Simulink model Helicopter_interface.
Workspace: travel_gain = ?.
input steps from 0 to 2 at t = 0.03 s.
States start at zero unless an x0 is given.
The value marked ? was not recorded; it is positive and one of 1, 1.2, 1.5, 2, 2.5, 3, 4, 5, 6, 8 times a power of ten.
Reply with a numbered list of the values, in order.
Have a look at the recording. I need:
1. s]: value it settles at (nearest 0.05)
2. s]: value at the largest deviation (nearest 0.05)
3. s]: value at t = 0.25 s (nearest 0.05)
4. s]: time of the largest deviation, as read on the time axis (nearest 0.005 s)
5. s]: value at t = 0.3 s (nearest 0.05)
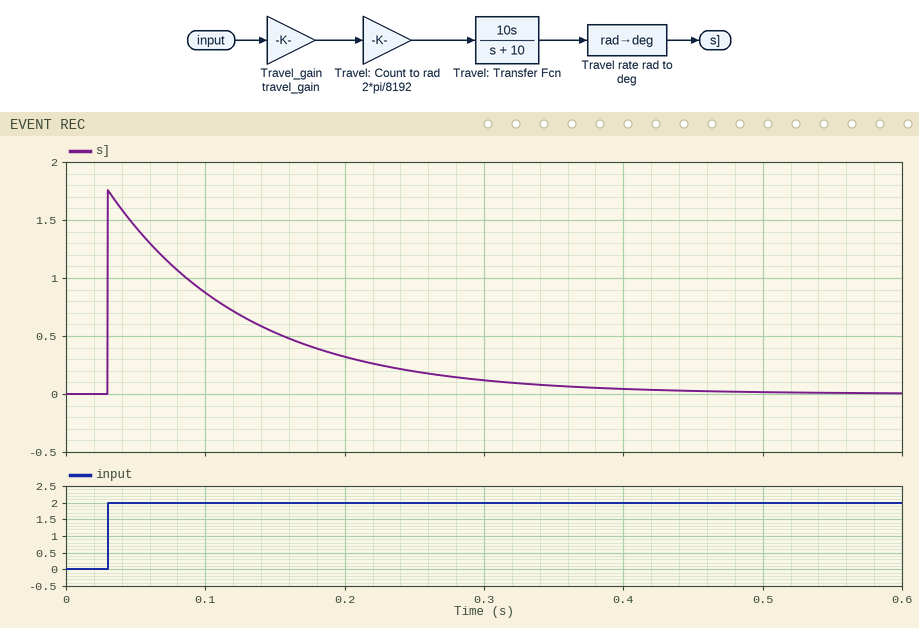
1. 0.00
2. 1.75
3. 0.20
4. 0.030 s
5. 0.10
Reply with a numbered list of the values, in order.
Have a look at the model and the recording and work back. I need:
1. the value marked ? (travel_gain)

1. 2
